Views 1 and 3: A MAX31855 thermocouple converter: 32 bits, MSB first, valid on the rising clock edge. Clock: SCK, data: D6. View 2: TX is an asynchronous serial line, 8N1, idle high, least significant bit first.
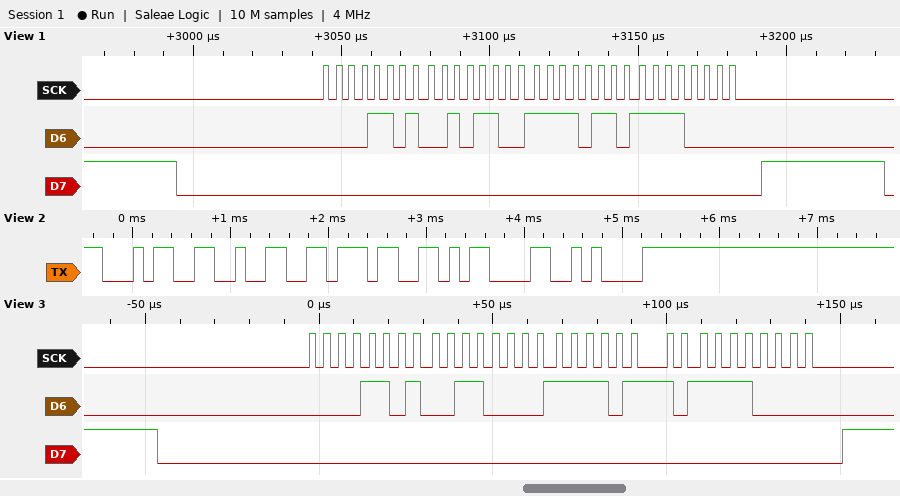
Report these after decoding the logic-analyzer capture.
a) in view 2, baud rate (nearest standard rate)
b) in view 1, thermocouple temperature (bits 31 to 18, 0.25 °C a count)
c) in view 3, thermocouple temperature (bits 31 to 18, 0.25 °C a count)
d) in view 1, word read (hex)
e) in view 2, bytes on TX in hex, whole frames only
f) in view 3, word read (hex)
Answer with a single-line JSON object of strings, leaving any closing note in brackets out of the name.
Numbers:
{"in view 2, baud rate": "9600 baud", "in view 1, thermocouple temperature": "210.75 °C", "in view 3, thermocouple temperature": "211.00 °C", "in view 1, word read": "0x0D2CF6F0", "in view 2, bytes on TX in hex, whole frames only": "34 32 37 0D 0A", "in view 3, word read": "0x0D30F6F0"}
